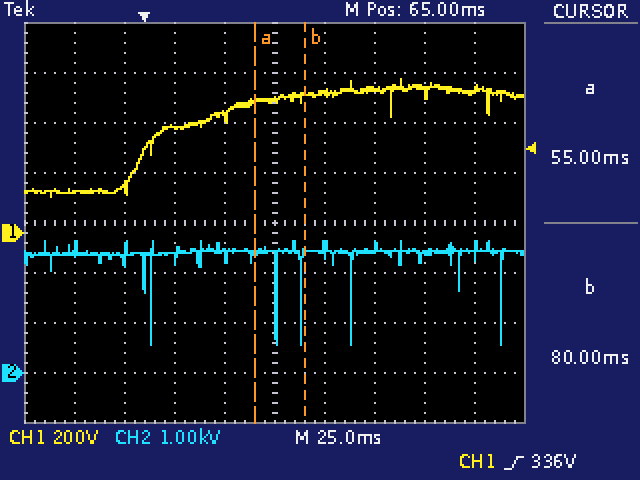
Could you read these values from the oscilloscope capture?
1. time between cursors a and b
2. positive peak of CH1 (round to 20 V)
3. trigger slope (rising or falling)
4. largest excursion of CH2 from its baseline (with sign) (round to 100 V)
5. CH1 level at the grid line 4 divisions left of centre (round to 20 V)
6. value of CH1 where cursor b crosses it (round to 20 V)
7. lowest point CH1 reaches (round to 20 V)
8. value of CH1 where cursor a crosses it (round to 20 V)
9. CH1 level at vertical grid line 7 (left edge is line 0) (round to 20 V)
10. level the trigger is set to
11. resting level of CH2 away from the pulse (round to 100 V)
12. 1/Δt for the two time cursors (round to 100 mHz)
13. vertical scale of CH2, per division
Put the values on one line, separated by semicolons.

25.0 ms; 620 V; rising; -1.9 kV; 160 V; 540 V; 140 V; 520 V; 580 V; 336 V; 2.4 kV; 40.0 Hz; 1 kV
